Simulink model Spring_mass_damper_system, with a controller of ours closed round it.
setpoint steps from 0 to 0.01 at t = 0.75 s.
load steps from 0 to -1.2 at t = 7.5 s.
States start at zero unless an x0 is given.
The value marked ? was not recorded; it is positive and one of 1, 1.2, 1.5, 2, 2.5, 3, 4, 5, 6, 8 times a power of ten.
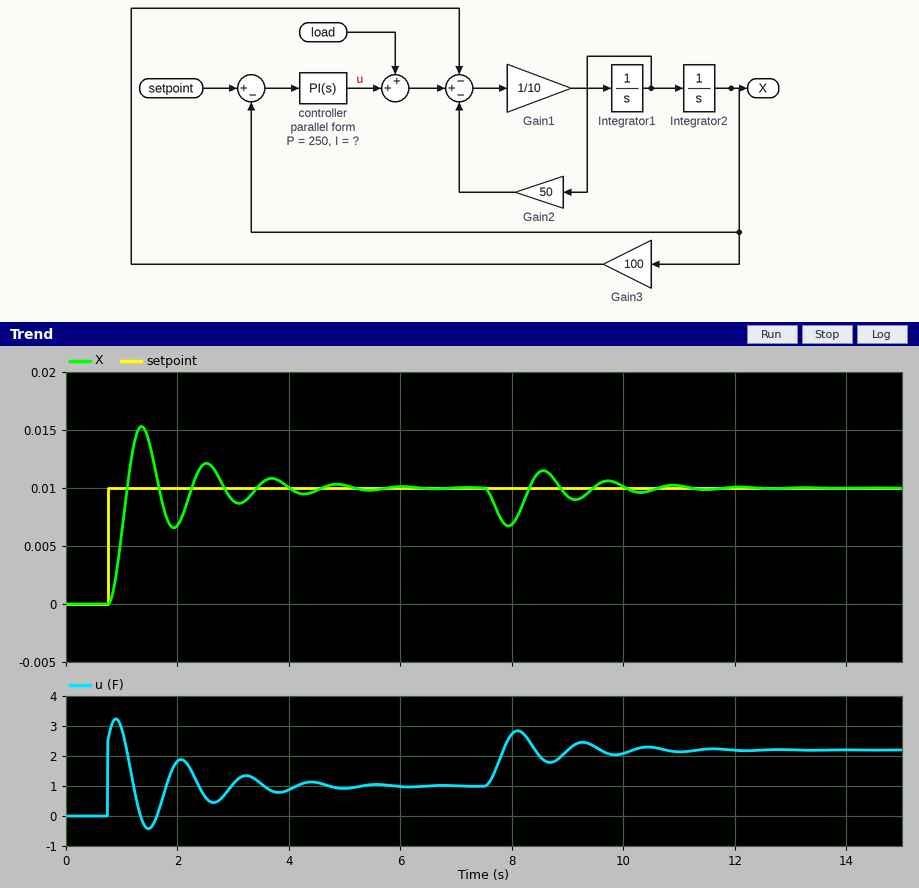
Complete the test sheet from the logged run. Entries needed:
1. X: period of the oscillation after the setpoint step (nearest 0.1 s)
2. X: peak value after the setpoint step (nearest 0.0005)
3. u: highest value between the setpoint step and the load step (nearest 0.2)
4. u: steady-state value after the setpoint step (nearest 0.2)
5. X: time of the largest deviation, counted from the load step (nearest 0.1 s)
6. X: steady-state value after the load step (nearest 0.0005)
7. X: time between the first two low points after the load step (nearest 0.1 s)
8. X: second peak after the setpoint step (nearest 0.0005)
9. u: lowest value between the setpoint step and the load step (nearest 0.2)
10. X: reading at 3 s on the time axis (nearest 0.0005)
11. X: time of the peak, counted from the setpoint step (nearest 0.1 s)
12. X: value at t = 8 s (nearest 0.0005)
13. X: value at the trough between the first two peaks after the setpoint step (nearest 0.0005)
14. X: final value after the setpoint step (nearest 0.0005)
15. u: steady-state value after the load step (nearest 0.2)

1.2 s
0.0155
3.2
1.0
0.4 s
0.0100
1.2 s
0.0120
-0.4
0.0090
0.6 s
0.0070
0.0065
0.0100
2.2
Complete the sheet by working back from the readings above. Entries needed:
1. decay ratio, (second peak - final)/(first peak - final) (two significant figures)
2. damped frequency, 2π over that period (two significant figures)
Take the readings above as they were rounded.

0.36
5.2 rad/s
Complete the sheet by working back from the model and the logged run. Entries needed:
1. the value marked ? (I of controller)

1000
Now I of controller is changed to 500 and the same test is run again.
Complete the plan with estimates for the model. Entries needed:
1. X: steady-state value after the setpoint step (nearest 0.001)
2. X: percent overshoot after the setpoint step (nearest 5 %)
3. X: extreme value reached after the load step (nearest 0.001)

0.010
25 %
0.006
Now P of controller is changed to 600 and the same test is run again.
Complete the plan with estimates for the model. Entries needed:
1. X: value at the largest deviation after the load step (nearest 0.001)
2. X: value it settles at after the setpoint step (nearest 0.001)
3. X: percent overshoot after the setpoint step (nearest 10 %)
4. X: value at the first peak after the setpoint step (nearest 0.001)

0.008
0.010
40 %
0.014
